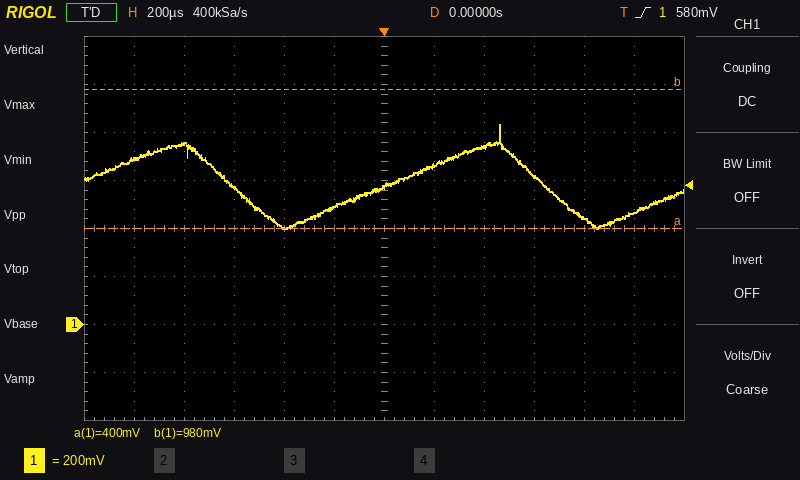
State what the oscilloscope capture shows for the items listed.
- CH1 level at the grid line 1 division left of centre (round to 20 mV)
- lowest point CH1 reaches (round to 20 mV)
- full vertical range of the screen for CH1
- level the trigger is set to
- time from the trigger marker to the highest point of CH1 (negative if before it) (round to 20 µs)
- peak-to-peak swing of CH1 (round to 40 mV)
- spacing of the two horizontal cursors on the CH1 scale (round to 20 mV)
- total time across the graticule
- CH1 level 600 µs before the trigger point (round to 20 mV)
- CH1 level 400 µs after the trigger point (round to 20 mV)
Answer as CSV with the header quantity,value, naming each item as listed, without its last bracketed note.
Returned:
quantity,value
CH1 level at the grid line 1 division left of centre,500 mV
lowest point CH1 reaches,400 mV
full vertical range of the screen for CH1,1.6 V
level the trigger is set to,580 mV
time from the trigger marker to the highest point of CH1 (negative if before it),+460 µs
peak-to-peak swing of CH1,440 mV
spacing of the two horizontal cursors on the CH1 scale,580 mV
total time across the graticule,2.4 ms
CH1 level 600 µs before the trigger point,580 mV
CH1 level 400 µs after the trigger point,740 mV
